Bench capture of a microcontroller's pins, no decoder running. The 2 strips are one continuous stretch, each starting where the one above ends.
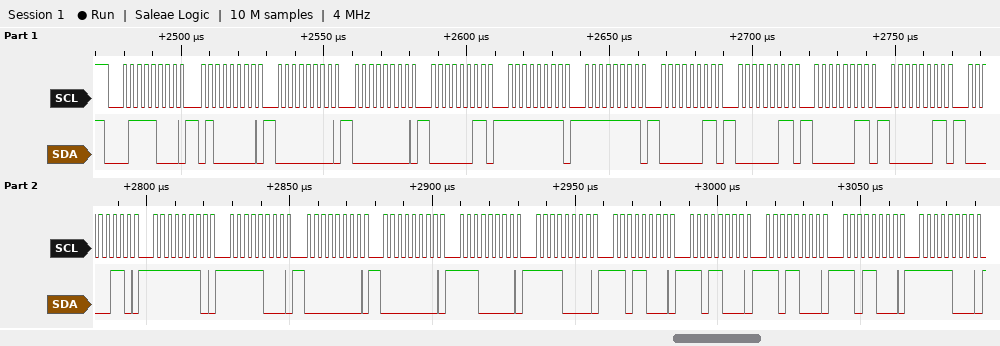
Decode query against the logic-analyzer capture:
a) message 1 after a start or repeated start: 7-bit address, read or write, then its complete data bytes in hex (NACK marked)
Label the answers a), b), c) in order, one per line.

a) 0x3C write: 40 00 00 03 FF FF 03 03 03 03 06 FE F8 00 00 E0 F0 D8 D8 D8 D8 F8
